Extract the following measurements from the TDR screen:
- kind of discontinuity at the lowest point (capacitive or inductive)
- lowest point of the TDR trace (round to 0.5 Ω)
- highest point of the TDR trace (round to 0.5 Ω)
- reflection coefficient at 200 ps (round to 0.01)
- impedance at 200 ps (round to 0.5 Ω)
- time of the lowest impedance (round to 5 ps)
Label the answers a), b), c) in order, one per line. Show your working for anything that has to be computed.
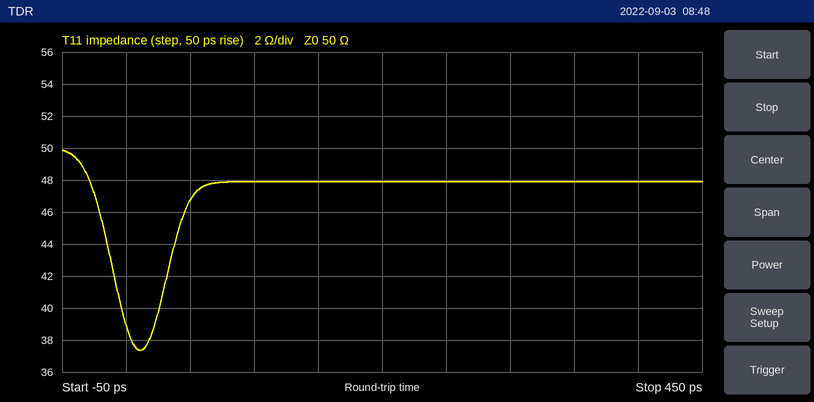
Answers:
a) capacitive
b) 37.5 Ω
c) 50.0 Ω
d) (48 − 50)/(48 + 50) ≈ -0.02
e) 48.0 Ω
f) 10 ps
